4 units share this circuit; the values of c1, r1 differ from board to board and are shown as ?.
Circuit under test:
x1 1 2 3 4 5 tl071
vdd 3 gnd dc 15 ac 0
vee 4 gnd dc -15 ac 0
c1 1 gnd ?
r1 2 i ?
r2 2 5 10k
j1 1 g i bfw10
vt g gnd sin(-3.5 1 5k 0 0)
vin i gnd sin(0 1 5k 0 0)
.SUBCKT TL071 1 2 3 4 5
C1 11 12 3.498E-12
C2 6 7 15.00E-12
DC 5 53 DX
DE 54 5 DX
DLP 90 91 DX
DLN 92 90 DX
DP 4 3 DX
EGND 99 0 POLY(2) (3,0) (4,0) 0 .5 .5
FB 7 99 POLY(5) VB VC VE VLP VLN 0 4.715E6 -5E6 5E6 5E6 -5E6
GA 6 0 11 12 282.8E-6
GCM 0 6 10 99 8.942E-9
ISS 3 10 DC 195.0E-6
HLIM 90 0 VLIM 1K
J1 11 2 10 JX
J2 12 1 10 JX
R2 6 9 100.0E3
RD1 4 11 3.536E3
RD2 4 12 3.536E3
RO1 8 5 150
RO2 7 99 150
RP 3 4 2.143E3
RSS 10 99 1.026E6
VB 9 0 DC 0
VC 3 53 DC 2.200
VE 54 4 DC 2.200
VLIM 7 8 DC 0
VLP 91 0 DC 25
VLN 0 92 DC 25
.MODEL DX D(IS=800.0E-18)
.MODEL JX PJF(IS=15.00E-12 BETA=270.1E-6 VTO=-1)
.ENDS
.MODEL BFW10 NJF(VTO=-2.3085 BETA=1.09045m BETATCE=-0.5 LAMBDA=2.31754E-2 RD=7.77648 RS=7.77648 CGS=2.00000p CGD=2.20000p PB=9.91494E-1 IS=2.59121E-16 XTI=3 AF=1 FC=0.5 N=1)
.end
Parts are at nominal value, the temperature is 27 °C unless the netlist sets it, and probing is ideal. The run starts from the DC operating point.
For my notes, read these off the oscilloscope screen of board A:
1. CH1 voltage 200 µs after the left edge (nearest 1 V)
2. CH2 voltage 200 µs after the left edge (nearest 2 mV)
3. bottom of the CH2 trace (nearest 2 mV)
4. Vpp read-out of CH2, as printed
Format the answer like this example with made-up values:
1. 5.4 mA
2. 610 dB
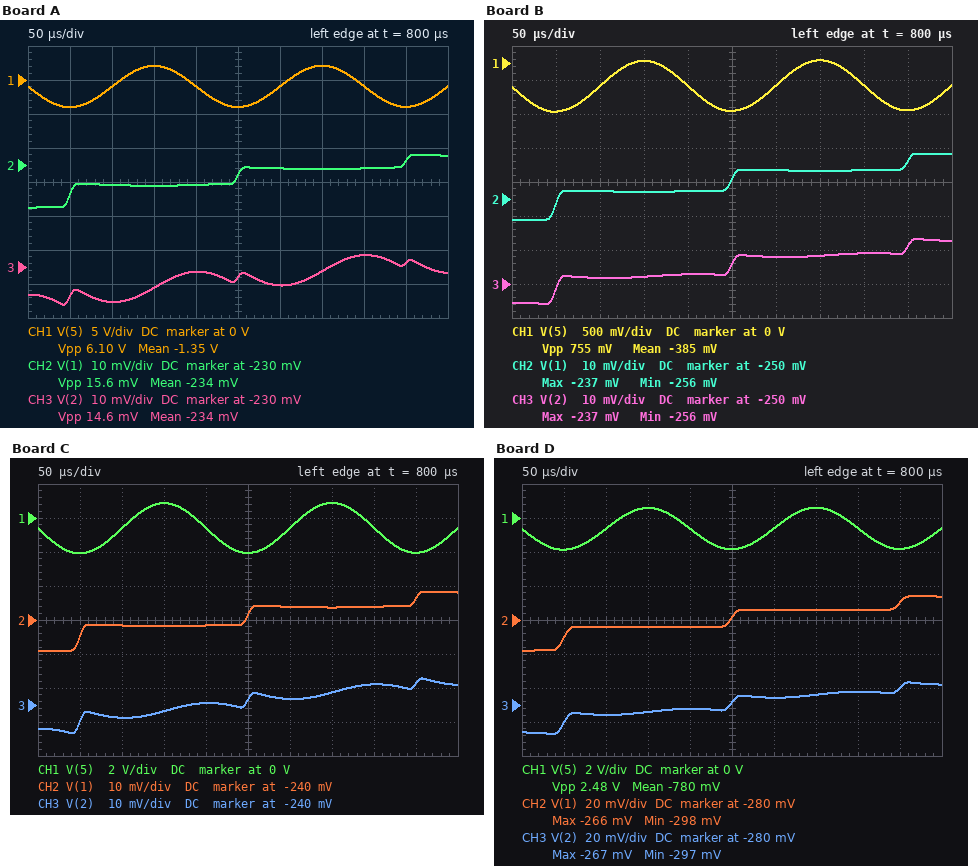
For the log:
1. -1 V
2. -236 mV
3. -242 mV
4. 15.6 mV
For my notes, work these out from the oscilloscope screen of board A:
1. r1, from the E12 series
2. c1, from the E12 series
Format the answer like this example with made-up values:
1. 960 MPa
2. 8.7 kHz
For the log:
1. 3.3 kΩ
2. 3.9 nF
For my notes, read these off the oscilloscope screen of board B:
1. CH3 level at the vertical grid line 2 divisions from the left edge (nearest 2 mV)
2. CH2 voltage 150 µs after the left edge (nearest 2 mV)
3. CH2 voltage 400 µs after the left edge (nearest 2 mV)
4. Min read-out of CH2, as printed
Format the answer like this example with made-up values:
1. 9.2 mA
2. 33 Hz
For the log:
1. -248 mV
2. -248 mV
3. -242 mV
4. -256 mV
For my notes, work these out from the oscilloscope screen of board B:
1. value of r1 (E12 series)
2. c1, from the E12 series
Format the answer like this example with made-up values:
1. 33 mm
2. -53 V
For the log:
1. 27 kΩ
2. 5.6 nF
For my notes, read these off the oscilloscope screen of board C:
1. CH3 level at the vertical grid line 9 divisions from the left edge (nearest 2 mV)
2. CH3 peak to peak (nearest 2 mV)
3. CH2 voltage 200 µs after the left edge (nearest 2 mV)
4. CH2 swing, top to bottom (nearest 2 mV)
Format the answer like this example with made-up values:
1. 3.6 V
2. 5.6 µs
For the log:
1. -234 mV
2. 16 mV
3. -242 mV
4. 18 mV
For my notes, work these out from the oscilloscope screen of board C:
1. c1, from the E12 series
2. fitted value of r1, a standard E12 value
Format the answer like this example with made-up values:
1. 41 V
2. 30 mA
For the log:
1. 4.7 nF
2. 6.8 kΩ
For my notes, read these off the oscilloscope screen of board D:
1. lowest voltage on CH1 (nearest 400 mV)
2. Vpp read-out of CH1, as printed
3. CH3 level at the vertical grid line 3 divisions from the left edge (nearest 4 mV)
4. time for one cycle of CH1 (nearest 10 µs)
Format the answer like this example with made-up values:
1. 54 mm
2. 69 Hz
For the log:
1. -2.0 V
2. 2.48 V
3. -284 mV
4. 200 µs
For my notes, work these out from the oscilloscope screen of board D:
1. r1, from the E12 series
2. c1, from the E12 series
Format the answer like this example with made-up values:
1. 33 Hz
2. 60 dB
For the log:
1. 8.2 kΩ
2. 12 nF
